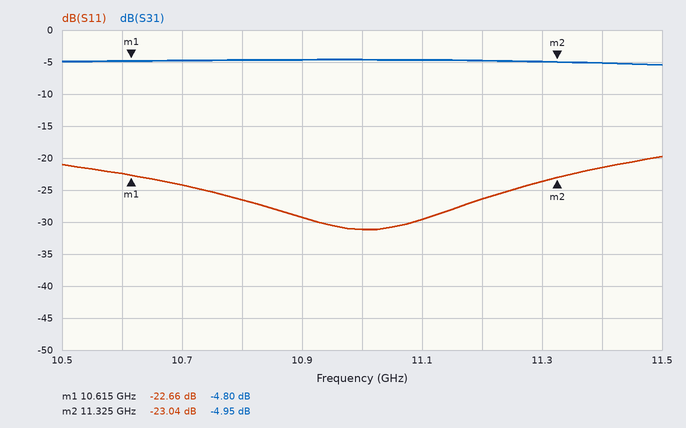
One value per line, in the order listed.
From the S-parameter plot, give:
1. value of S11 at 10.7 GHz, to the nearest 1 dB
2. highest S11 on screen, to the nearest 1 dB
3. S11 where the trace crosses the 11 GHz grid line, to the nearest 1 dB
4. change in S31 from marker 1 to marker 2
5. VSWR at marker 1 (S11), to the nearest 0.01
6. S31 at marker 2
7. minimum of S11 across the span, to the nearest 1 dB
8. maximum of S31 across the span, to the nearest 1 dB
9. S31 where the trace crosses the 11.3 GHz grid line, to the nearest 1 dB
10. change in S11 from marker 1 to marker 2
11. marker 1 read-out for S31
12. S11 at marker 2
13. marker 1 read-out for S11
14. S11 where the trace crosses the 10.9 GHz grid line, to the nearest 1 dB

-24 dB
-20 dB
-31 dB
-0.15 dB
1.16
-4.95 dB
-31 dB
-5 dB
-5 dB
-0.38 dB
-4.80 dB
-23.04 dB
-22.66 dB
-29 dB
